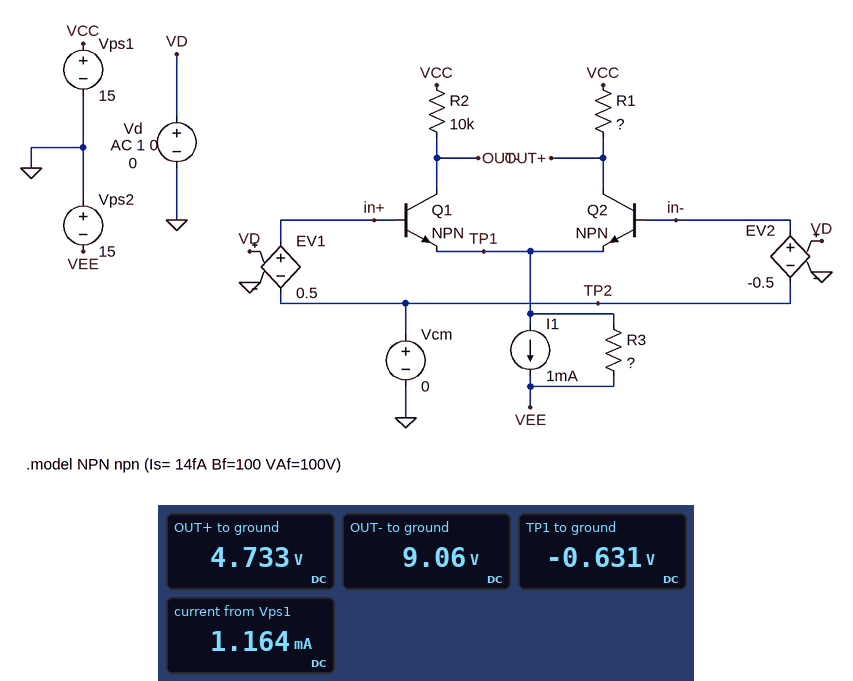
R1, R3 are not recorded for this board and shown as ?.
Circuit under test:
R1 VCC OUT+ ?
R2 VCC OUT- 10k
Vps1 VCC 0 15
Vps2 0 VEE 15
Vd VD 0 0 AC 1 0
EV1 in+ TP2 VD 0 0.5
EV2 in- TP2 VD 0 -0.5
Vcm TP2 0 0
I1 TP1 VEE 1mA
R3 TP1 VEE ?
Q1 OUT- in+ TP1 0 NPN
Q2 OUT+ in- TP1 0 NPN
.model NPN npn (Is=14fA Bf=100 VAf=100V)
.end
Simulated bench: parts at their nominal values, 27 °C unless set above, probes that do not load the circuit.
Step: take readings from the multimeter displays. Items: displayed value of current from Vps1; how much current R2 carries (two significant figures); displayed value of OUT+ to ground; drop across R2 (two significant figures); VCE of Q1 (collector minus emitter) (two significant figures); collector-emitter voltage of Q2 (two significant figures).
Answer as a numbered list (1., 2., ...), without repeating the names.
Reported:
1. 1.164 mA
2. 590 µA
3. 4.733 V
4. 5.9 V
5. 9.7 V
6. 5.4 V
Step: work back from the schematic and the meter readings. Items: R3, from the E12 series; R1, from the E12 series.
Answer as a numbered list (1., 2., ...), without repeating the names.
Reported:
1. 82 kΩ
2. 18 kΩ
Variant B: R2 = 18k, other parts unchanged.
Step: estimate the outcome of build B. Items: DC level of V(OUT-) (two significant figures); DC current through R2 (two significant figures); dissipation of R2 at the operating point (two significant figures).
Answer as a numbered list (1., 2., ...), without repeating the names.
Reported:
1. 4.5 V
2. 580 µA
3. 6.1 mW
